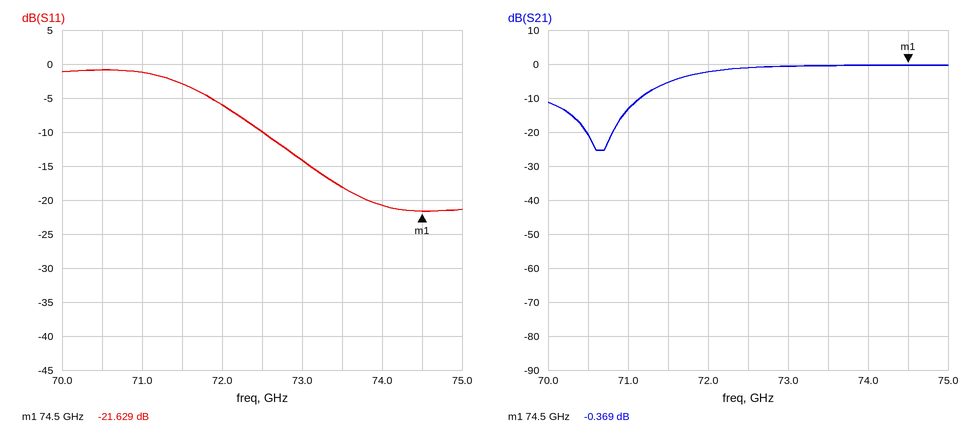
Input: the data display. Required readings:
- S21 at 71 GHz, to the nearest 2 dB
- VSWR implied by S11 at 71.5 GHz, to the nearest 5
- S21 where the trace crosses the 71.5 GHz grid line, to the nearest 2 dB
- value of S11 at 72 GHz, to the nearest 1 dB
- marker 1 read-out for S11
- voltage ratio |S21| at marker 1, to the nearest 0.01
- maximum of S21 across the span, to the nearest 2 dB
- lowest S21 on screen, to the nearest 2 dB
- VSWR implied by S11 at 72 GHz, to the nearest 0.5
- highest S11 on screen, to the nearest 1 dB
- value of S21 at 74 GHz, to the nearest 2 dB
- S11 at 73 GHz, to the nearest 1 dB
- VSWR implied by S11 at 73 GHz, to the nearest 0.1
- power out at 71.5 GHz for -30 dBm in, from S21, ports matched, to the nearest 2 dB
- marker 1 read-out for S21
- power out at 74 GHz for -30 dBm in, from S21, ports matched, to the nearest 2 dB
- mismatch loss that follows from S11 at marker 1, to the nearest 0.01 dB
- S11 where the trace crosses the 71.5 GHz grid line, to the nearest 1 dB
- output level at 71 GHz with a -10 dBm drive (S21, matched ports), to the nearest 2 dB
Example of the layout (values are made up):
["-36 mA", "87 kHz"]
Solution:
["-14 dB", "5", "-6 dB", "-6 dB", "-21.629 dB", "0.96", "0 dB", "-26 dB", "3.0", "-1 dB", "0 dB", "-14 dB", "1.5", "-36 dBm", "-0.369 dB", "-30 dBm", "0.03 dB", "-3 dB", "-24 dBm"]
